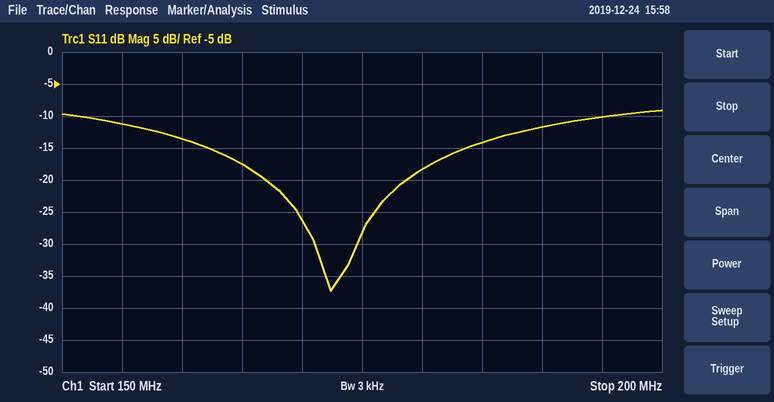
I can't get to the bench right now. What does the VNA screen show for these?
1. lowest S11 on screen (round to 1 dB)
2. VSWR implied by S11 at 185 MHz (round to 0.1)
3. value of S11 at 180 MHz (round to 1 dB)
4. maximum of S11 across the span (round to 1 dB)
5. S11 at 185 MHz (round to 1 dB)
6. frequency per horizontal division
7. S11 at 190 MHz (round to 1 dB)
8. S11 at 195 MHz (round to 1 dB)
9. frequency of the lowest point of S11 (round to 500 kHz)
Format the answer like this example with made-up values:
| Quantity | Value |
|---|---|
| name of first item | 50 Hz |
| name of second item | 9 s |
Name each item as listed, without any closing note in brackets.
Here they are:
| Quantity | Value |
|---|---|
| lowest S11 on screen | -37 dB |
| VSWR implied by S11 at 185 MHz | 1.5 |
| value of S11 at 180 MHz | -18 dB |
| maximum of S11 across the span | -9 dB |
| S11 at 185 MHz | -14 dB |
| frequency per horizontal division | 5 MHz |
| S11 at 190 MHz | -12 dB |
| S11 at 195 MHz | -10 dB |
| frequency of the lowest point of S11 | 172.5 MHz |
